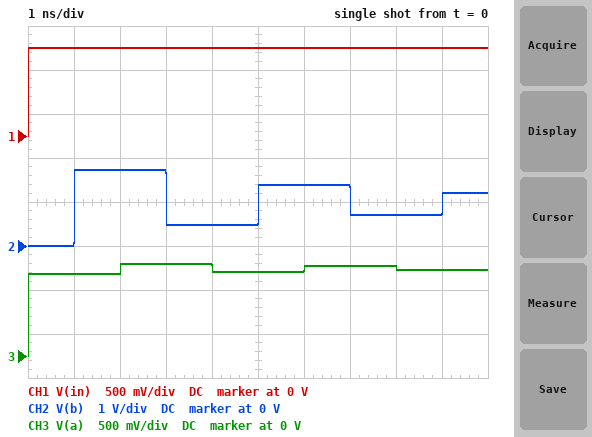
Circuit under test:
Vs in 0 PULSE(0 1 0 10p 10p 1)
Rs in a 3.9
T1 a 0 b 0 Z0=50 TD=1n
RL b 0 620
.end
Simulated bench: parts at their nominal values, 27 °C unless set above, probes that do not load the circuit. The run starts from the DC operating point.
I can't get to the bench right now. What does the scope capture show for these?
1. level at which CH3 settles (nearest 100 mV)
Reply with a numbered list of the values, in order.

1. 1.0 V
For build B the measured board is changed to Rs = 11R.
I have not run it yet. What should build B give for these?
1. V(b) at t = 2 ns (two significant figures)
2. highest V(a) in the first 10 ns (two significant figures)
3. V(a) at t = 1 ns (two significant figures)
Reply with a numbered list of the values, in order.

1. 1.5 V
2. 1.1 V
3. 820 mV
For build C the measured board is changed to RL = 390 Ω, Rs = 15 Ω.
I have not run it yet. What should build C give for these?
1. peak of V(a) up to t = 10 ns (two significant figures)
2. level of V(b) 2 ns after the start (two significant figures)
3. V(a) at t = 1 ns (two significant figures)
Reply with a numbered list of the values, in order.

1. 1.0 V
2. 1.4 V
3. 770 mV
